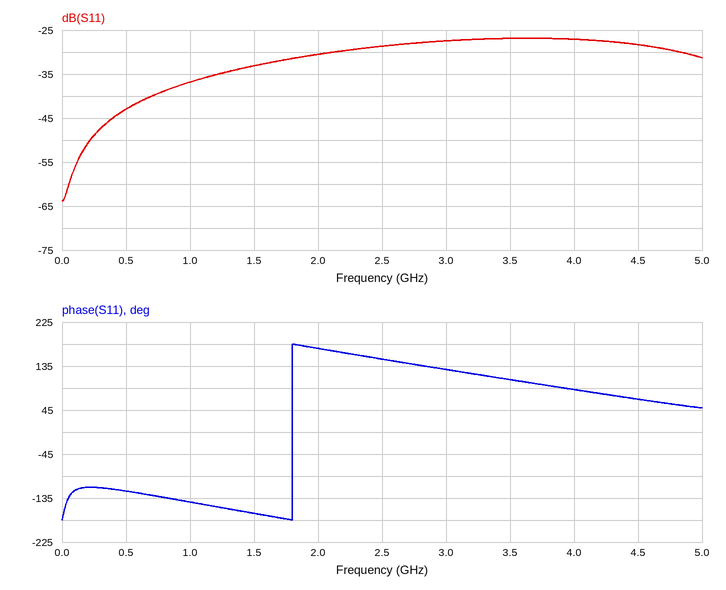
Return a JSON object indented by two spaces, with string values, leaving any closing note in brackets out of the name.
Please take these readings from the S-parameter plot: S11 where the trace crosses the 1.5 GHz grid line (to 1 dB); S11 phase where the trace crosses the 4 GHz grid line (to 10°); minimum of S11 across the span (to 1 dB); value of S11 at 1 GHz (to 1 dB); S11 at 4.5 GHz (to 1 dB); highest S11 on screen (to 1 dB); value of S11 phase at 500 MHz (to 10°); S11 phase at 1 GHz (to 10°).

{
  "S11 where the trace crosses the 1.5 GHz grid line": "-33 dB",
  "S11 phase where the trace crosses the 4 GHz grid line": "90°",
  "minimum of S11 across the span": "-64 dB",
  "value of S11 at 1 GHz": "-37 dB",
  "S11 at 4.5 GHz": "-28 dB",
  "highest S11 on screen": "-27 dB",
  "value of S11 phase at 500 MHz": "-120°",
  "S11 phase at 1 GHz": "-140°"
}
